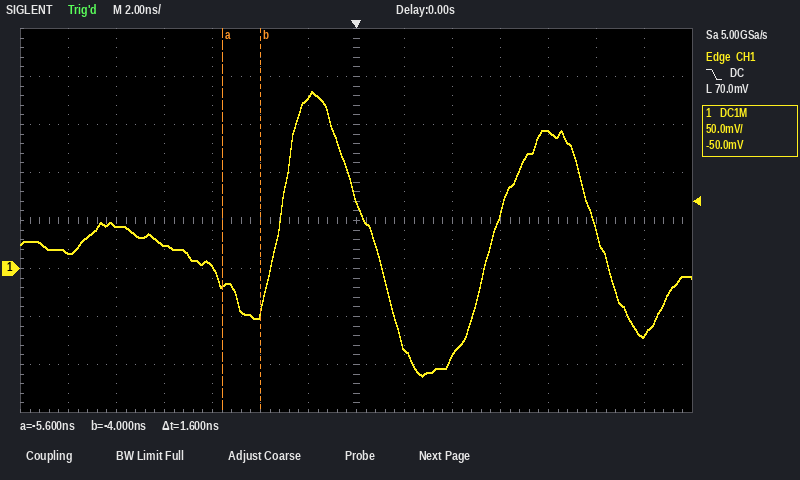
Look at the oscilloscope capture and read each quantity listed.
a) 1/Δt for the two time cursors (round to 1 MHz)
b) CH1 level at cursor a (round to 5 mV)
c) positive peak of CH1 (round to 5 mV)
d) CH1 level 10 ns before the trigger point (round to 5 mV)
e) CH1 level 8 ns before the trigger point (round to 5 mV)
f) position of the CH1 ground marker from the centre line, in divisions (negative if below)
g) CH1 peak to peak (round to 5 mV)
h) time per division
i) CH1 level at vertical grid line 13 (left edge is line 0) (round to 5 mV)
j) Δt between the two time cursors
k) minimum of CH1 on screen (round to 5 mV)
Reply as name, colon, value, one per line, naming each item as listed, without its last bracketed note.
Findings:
1/Δt for the two time cursors: 625 MHz
CH1 level at cursor a: -15 mV
positive peak of CH1: 185 mV
CH1 level 10 ns before the trigger point: 45 mV
CH1 level 8 ns before the trigger point: 25 mV
position of the CH1 ground marker from the centre line, in divisions: -1.0 div
CH1 peak to peak: 295 mV
time per division: 2 ns
CH1 level at vertical grid line 13 (left edge is line 0): -70 mV
Δt between the two time cursors: 1.6 ns
minimum of CH1 on screen: -110 mV
